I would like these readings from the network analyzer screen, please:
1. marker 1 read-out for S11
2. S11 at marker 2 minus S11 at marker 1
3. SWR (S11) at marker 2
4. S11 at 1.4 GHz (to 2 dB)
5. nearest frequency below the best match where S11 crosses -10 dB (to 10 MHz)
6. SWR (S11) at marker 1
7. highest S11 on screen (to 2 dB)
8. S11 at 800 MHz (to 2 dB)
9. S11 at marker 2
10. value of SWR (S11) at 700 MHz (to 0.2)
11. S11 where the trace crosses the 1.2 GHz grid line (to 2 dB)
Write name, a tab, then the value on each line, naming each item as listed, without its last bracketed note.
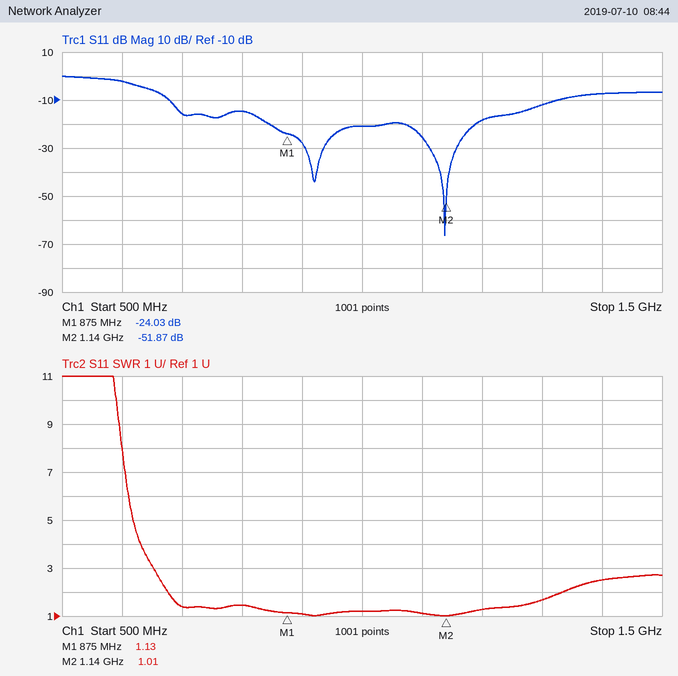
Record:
marker 1 read-out for S11	-24.03 dB
S11 at marker 2 minus S11 at marker 1	-27.84 dB
SWR (S11) at marker 2	1.01
S11 at 1.4 GHz	-8 dB
nearest frequency below the best match where S11 crosses -10 dB	680 MHz
SWR (S11) at marker 1	1.13
highest S11 on screen	0 dB
S11 at 800 MHz	-14 dB
S11 at marker 2	-51.87 dB
value of SWR (S11) at 700 MHz	1.4
S11 where the trace crosses the 1.2 GHz grid line	-18 dB
